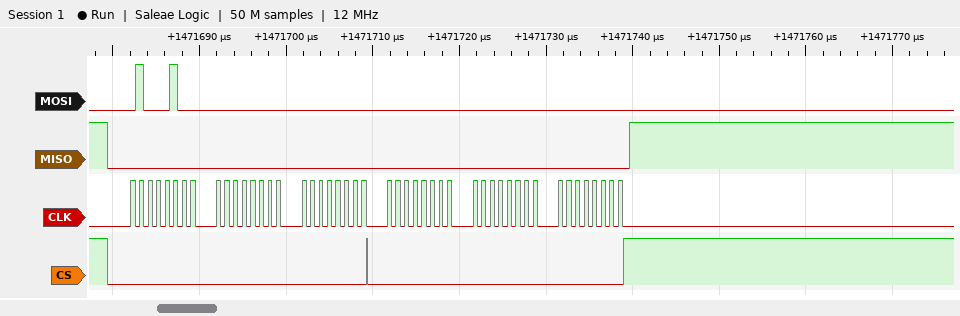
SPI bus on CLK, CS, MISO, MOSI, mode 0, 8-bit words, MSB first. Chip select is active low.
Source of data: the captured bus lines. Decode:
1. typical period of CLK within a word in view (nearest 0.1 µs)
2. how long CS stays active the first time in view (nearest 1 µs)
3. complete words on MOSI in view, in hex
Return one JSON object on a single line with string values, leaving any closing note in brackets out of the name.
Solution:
{"typical period of CLK within a word in view": "1 µs", "how long CS stays active the first time in view": "30 µs", "complete words on MOSI in view, in hex": "44, 00, 00, 00, 00, 00"}
